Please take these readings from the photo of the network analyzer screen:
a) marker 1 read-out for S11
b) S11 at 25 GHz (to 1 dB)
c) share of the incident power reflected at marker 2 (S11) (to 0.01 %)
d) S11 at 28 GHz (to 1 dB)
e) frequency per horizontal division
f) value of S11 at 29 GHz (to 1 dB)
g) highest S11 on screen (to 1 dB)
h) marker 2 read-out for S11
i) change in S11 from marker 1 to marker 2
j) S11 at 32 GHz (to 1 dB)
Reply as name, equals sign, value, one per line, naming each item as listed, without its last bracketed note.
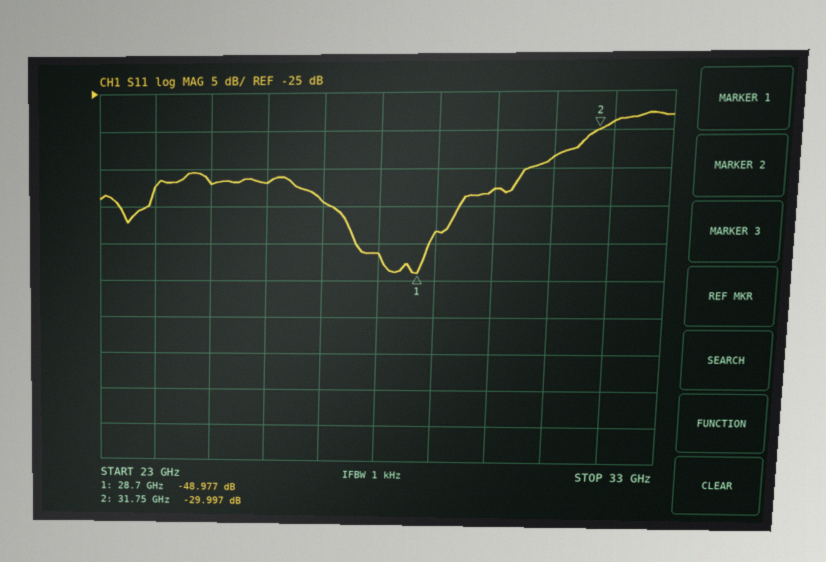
marker 1 read-out for S11 = -48.977 dB
S11 at 25 GHz = -37 dB
share of the incident power reflected at marker 2 (S11) = 0.10 %
S11 at 28 GHz = -46 dB
frequency per horizontal division = 1 GHz
value of S11 at 29 GHz = -43 dB
highest S11 on screen = -28 dB
marker 2 read-out for S11 = -29.997 dB
change in S11 from marker 1 to marker 2 = 18.980 dB
S11 at 32 GHz = -29 dB
